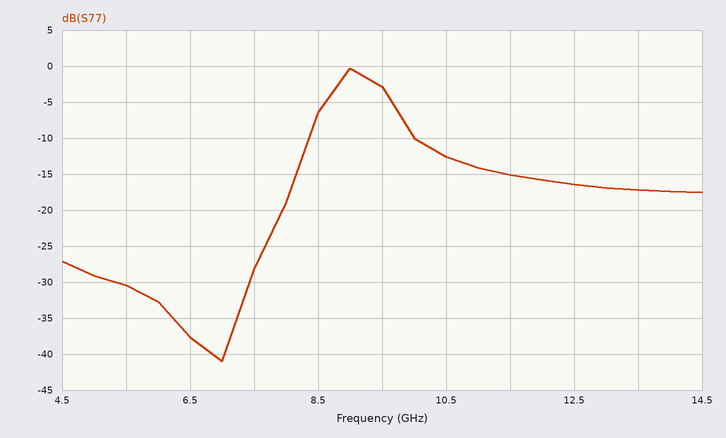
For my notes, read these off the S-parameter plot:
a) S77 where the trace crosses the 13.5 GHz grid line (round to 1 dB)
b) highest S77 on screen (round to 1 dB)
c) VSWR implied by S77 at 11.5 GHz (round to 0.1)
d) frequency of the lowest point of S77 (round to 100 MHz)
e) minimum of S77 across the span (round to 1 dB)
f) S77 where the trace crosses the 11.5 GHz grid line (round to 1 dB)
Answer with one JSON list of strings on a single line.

["-17 dB", "0 dB", "1.4", "7.0 GHz", "-41 dB", "-15 dB"]
